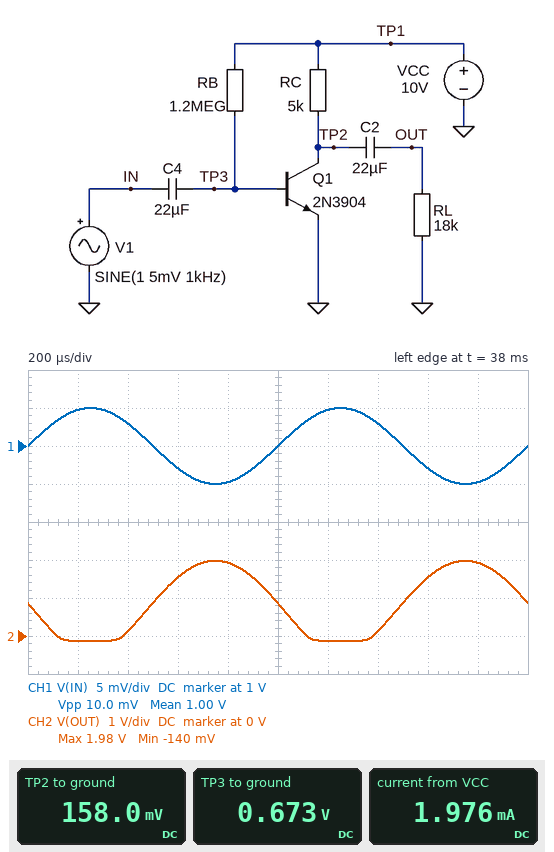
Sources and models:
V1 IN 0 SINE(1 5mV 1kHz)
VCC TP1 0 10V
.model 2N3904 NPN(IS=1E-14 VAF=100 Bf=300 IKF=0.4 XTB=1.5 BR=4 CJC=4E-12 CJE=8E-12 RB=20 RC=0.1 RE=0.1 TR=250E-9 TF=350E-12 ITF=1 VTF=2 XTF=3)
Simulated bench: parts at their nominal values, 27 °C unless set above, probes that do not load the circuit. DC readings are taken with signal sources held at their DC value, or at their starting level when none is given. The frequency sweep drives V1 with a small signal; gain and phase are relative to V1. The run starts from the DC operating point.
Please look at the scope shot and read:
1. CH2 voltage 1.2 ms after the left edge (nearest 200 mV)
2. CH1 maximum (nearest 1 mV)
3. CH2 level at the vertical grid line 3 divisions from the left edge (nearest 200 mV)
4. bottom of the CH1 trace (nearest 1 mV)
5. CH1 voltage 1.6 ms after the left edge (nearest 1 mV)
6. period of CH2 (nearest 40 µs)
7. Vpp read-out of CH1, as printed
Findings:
-200 mV
1.005 V
1.6 V
995 mV
997 mV
1.00 ms
10.0 mV
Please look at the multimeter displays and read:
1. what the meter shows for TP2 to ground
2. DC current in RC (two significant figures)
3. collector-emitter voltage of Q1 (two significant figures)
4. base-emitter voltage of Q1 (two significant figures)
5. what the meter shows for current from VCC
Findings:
158.0 mV
2.0 mA
160 mV
670 mV
1.976 mA
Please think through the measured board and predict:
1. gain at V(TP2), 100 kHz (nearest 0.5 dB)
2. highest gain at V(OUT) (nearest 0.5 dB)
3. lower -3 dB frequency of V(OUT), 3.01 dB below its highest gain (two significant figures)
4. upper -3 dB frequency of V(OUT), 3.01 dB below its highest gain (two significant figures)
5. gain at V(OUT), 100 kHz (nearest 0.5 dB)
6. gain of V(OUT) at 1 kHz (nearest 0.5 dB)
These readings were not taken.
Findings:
42.5 dB
42.5 dB
44 Hz
720 kHz
42.5 dB
42.5 dB
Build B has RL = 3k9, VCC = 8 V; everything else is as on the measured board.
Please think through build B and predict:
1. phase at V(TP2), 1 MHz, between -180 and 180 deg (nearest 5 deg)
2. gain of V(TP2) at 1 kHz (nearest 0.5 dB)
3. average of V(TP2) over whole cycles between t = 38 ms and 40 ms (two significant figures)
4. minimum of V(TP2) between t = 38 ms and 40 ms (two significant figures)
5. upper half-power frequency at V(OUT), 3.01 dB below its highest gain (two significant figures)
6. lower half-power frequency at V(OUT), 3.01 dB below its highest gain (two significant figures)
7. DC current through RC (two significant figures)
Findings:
140 deg
39.0 dB
600 mV
100 mV
1.3 MHz
22 Hz
1.6 mA
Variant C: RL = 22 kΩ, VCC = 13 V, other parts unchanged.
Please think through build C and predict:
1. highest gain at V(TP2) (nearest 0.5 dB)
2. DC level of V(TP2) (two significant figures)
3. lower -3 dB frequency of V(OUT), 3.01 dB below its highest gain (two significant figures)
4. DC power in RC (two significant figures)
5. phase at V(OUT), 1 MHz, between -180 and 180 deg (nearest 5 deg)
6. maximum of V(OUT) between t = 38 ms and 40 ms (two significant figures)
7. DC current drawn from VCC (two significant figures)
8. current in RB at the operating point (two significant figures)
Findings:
43.0 dB
160 mV
64 Hz
33 mW
120 deg
2.6 V
2.6 mA
10 µA
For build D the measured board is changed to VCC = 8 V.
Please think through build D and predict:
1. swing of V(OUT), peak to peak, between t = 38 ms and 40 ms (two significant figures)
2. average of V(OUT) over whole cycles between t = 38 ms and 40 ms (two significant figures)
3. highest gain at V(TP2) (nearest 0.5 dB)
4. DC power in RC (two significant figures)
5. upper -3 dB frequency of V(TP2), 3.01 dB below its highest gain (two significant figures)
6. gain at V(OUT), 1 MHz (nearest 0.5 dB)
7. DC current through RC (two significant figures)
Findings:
1.7 V
700 mV
42.0 dB
12 mW
900 kHz
38.5 dB
1.6 mA
